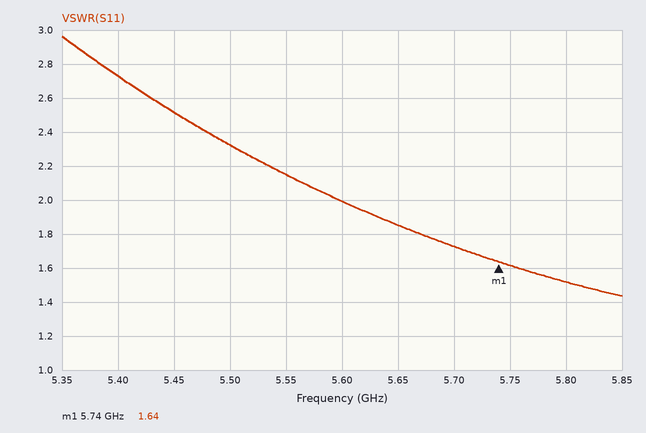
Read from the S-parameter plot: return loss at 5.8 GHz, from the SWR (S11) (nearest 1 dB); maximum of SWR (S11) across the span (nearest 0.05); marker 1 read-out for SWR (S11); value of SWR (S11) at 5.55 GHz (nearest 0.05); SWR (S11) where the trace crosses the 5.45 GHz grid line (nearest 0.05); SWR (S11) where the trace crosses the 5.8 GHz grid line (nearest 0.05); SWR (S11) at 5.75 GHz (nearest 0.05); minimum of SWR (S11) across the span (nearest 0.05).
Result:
14 dB
2.95
1.64
2.15
2.50
1.50
1.60
1.45
